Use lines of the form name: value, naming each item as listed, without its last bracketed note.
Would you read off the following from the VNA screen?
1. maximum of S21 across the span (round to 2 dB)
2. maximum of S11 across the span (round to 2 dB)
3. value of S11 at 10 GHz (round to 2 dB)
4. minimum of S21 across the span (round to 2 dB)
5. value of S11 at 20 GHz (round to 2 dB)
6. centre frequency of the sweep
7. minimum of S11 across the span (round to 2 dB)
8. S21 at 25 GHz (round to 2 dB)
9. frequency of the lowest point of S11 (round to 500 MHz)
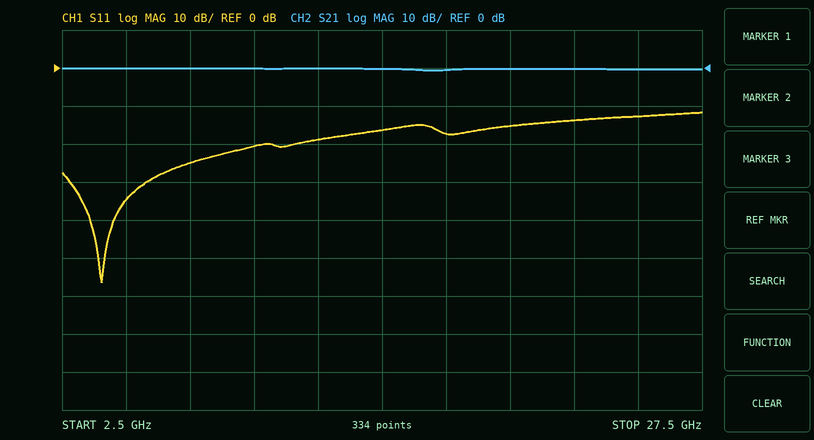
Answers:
maximum of S21 across the span: 0 dB
maximum of S11 across the span: -12 dB
value of S11 at 10 GHz: -20 dB
minimum of S21 across the span: 0 dB
value of S11 at 20 GHz: -16 dB
centre frequency of the sweep: 15 GHz
minimum of S11 across the span: -56 dB
S21 at 25 GHz: 0 dB
frequency of the lowest point of S11: 4.0 GHz
